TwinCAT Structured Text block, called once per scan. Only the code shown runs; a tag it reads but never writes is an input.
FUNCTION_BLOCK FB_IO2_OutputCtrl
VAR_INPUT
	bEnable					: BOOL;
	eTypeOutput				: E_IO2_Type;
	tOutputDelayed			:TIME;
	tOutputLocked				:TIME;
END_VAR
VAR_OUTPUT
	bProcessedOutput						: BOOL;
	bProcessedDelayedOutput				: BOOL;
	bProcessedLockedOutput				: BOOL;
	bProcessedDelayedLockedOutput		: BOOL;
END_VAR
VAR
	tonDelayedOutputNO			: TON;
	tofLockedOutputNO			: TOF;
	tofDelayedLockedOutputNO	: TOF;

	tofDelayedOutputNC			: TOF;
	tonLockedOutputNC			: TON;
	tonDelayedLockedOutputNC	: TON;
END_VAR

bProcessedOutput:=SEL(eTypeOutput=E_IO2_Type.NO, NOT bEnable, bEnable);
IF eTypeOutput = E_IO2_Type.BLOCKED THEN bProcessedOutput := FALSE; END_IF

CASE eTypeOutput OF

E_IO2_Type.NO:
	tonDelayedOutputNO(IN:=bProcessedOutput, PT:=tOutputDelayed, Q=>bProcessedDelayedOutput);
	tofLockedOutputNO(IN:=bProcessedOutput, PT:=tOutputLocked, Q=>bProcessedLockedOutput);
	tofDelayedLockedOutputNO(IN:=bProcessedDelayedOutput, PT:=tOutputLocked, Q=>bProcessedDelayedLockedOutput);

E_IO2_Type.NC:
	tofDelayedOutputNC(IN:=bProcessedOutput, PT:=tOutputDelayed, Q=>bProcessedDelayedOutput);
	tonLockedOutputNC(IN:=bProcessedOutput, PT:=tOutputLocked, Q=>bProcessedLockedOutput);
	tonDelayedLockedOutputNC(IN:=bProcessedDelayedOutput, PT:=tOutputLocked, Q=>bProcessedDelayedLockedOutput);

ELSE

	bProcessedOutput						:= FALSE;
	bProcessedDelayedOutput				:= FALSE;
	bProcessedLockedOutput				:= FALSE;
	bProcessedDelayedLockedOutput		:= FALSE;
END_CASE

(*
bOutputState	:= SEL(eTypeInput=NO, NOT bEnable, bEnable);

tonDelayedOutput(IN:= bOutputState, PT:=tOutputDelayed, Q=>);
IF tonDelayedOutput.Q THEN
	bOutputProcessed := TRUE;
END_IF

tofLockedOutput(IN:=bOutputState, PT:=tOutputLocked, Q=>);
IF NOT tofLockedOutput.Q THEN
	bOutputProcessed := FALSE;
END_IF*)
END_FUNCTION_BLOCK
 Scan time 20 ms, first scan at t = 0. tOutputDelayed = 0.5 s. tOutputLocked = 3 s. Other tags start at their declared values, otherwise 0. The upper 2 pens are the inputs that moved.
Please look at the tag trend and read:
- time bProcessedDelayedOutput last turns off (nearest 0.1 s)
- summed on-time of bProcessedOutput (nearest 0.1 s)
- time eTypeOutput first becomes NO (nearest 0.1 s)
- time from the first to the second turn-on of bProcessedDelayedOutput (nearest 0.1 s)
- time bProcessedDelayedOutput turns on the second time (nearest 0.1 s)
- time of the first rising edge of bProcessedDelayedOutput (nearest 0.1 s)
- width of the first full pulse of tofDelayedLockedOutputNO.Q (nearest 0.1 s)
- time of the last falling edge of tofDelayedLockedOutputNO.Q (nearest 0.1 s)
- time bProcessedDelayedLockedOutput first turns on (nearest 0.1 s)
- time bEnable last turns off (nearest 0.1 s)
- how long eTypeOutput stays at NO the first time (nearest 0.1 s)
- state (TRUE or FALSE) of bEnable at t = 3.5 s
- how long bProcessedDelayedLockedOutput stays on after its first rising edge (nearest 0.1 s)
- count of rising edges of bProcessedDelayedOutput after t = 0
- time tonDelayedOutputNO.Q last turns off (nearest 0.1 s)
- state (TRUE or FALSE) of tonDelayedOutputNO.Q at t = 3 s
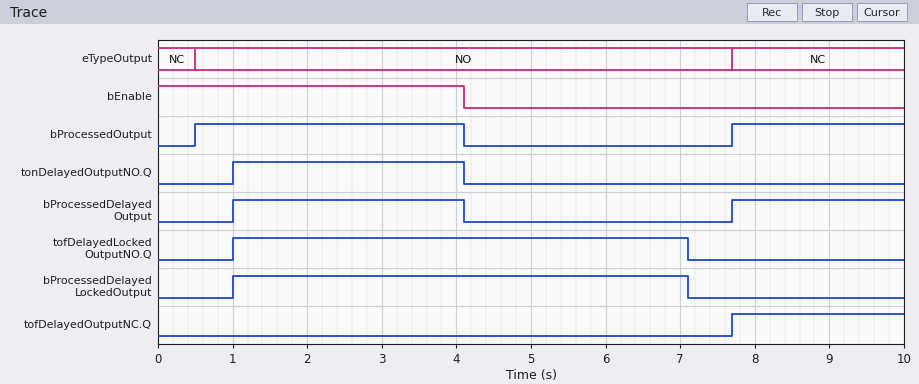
4.1 s
5.9 s
0.5 s
6.7 s
7.7 s
1.0 s
6.1 s
7.1 s
1.0 s
4.1 s
7.2 s
TRUE
6.1 s
2
4.1 s
TRUE
